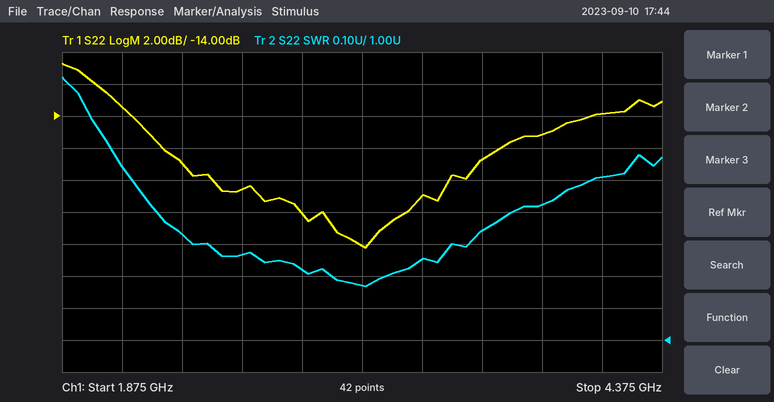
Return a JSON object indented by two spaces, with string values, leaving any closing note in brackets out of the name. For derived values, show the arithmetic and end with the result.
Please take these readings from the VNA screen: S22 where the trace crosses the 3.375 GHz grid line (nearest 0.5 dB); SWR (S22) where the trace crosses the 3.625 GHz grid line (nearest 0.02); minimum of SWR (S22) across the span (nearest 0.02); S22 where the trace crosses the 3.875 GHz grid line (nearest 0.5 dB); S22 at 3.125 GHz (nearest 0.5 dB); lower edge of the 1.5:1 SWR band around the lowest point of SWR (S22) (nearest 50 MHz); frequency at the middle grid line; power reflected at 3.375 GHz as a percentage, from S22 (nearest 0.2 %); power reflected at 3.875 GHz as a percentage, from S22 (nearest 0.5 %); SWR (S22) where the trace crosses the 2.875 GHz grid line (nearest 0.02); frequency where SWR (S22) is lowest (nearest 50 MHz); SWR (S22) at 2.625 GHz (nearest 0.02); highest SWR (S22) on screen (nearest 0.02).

{
  "S22 where the trace crosses the 3.375 GHz grid line": "-19.0 dB",
  "SWR (S22) where the trace crosses the 3.625 GHz grid line": "1.34",
  "minimum of SWR (S22) across the span": "1.16",
  "S22 where the trace crosses the 3.875 GHz grid line": "-15.0 dB",
  "S22 at 3.125 GHz": "-22.0 dB",
  "lower edge of the 1.5:1 SWR band around the lowest point of SWR (S22)": "2.15 GHz",
  "frequency at the middle grid line": "3.125 GHz",
  "power reflected at 3.375 GHz as a percentage, from S22": "10^(-19/10) ≈ 1.26 %, so 1.2 % to the nearest 0.2 %",
  "power reflected at 3.875 GHz as a percentage, from S22": "10^(-15/10) ≈ 3.16 %, so 3.0 % to the nearest 0.5 %",
  "SWR (S22) where the trace crosses the 2.875 GHz grid line": "1.22",
  "frequency where SWR (S22) is lowest": "3.15 GHz",
  "SWR (S22) at 2.625 GHz": "1.26",
  "highest SWR (S22) on screen": "1.82"
}
